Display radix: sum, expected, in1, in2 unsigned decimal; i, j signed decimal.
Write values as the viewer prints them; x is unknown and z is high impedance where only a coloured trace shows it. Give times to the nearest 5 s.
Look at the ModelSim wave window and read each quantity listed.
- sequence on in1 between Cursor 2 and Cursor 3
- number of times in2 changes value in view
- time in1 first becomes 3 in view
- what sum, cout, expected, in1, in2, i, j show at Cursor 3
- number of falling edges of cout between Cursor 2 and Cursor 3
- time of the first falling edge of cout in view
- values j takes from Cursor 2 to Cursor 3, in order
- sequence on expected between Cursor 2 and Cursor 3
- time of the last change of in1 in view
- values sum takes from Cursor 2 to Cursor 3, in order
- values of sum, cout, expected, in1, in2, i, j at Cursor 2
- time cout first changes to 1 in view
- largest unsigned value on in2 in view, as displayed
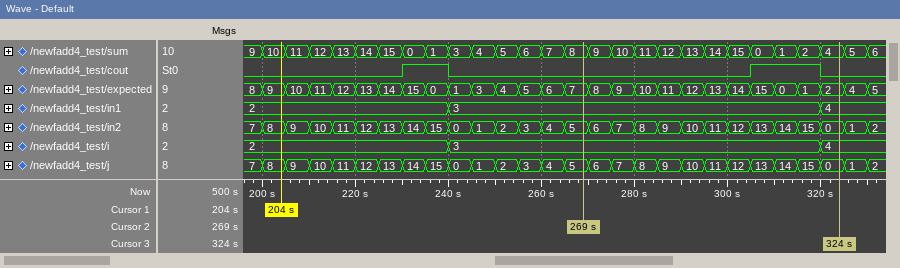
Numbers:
3, 4
27
240 s
sum=4, cout=0, expected=2, in1=4, in2=0, i=4, j=0
1
240 s
5, 6, 7, 8, 9, 10, 11, 12, 13, 14, 15, 0
7, 8, 9, 10, 11, 12, 13, 14, 15, 0, 1, 2
320 s
8, 9, 10, 11, 12, 13, 14, 15, 0, 1, 2, 4
sum=8, cout=0, expected=7, in1=3, in2=5, i=3, j=5
230 s
15
